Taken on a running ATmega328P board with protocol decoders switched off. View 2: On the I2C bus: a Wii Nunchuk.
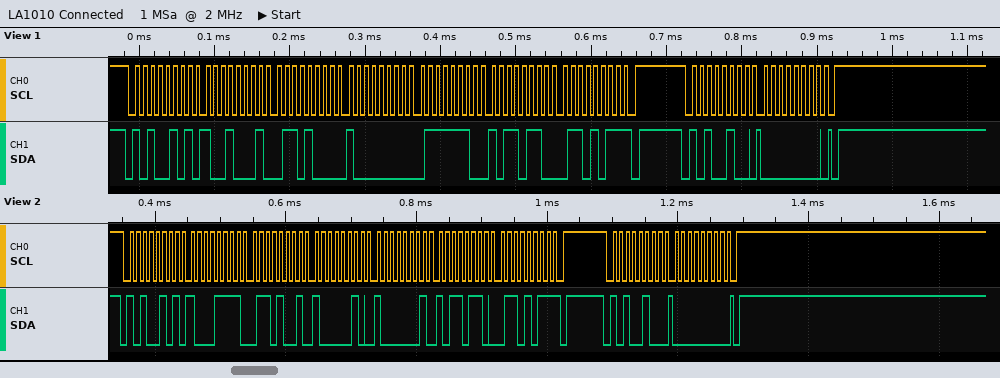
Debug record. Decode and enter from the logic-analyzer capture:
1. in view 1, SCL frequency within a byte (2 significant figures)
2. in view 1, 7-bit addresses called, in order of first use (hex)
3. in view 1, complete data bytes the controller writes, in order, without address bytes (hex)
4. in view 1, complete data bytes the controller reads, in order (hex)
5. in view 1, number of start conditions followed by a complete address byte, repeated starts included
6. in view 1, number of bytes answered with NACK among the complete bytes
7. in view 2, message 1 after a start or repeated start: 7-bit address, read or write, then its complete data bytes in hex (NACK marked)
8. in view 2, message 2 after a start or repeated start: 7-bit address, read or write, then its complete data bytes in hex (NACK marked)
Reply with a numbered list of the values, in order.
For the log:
1. 100 kHz
2. 0x52
3. 00
4. 91 68 80 7E B6 6B
5. 2
6. 1
7. 0x52 read: 8F 69 82 81 B6 6B NACK
8. 0x52 write: 00
